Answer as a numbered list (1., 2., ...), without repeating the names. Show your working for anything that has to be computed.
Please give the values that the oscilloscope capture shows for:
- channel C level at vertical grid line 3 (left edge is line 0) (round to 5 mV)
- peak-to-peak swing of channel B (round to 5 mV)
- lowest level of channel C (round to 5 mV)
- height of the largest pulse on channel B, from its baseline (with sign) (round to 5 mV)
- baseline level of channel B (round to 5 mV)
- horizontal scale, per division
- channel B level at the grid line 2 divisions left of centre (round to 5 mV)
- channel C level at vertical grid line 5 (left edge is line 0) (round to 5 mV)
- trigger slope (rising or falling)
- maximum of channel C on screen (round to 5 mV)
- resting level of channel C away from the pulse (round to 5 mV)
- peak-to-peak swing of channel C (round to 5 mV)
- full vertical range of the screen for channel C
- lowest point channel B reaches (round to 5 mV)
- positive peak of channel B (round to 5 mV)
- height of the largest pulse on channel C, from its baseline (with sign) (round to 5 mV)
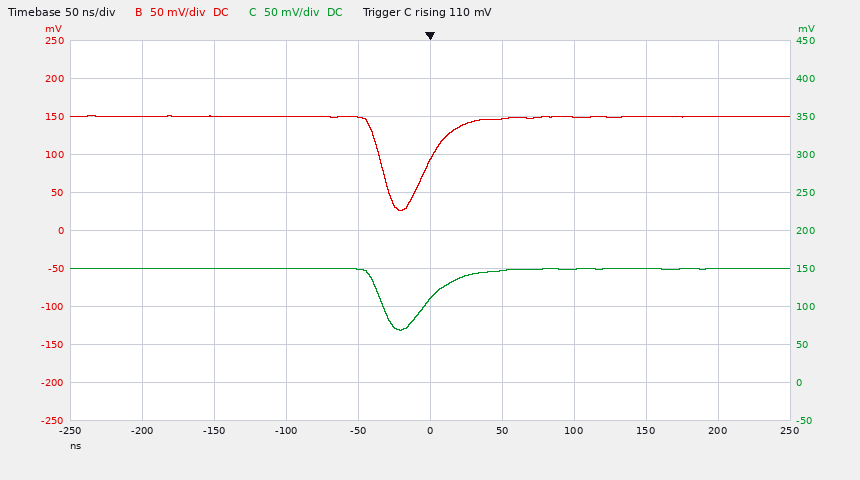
1. 150 mV
2. 150 mV − (25 mV) = 125 mV
3. 70 mV
4. 25 mV − (150 mV) = -125 mV
5. 150 mV
6. 50 ns
7. 150 mV
8. 110 mV
9. rising
10. 150 mV
11. 150 mV
12. 150 mV − (70 mV) = 80 mV
13. 500 mV
14. 25 mV
15. 150 mV
16. 70 mV − (150 mV) = -80 mV
